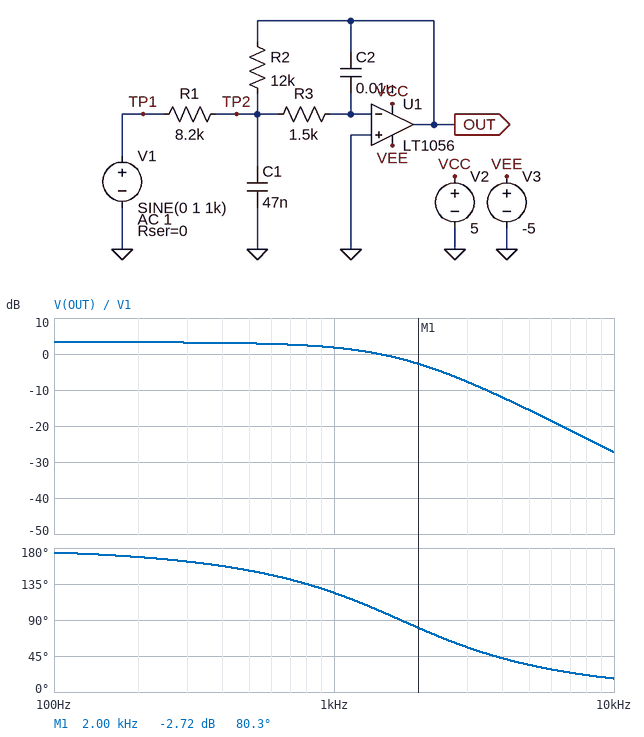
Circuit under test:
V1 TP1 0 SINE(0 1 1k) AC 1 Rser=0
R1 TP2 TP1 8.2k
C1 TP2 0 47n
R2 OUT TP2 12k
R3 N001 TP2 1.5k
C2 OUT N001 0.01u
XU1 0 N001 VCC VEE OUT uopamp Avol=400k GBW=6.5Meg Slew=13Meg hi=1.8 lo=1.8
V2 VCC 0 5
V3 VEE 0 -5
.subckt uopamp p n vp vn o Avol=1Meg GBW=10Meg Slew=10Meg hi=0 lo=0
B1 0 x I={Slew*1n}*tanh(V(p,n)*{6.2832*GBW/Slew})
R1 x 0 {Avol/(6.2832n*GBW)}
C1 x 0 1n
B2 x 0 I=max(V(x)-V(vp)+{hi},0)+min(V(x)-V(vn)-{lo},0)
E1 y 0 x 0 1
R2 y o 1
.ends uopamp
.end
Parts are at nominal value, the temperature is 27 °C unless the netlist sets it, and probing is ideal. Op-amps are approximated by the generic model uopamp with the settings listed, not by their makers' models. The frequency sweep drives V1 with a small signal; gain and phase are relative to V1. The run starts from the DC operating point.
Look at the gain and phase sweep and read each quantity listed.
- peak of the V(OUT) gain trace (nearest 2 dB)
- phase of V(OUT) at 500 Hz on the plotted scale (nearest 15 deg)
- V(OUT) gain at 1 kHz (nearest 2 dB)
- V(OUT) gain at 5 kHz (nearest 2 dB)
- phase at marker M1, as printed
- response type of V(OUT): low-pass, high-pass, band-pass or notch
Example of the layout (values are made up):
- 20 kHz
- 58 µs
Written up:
- 4 dB
- 150 deg
- 2 dB
- -16 dB
- 80.3 deg
- low-pass
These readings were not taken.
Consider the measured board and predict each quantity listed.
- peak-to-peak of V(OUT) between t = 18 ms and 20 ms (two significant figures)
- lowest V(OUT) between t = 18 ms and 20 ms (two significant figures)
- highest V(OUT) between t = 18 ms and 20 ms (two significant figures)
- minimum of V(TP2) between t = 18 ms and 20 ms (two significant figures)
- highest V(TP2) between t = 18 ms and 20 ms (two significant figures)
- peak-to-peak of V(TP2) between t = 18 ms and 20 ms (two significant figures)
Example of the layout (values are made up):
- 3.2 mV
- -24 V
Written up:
- 2.5 V
- -1.2 V
- 1.2 V
- -120 mV
- 120 mV
- 230 mV
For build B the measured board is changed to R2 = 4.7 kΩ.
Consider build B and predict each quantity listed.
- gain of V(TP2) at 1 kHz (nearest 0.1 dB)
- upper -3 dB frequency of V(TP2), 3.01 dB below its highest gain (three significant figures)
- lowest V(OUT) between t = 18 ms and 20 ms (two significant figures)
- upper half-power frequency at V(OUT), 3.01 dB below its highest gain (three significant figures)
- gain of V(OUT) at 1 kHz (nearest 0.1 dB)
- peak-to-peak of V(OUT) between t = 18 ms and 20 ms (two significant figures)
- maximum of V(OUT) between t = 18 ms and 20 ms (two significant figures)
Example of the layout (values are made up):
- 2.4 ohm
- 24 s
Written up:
- -25.1 dB
- 4.93 kHz
- -590 mV
- 3.05 kHz
- -4.6 dB
- 1.2 V
- 590 mV
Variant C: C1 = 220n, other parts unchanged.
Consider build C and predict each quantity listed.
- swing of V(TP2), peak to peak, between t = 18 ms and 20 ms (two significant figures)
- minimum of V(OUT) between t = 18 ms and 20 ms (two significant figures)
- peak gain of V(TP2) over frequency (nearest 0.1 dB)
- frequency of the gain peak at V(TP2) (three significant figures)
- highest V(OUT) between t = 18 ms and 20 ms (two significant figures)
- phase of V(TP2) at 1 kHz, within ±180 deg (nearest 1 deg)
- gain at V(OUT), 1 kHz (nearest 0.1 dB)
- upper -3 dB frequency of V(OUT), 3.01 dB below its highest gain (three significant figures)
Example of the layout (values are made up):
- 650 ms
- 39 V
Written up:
- 240 mV
- -1.3 V
- -17.1 dB
- 799 Hz
- 1.3 V
- -30 deg
- 2.2 dB
- 950 Hz
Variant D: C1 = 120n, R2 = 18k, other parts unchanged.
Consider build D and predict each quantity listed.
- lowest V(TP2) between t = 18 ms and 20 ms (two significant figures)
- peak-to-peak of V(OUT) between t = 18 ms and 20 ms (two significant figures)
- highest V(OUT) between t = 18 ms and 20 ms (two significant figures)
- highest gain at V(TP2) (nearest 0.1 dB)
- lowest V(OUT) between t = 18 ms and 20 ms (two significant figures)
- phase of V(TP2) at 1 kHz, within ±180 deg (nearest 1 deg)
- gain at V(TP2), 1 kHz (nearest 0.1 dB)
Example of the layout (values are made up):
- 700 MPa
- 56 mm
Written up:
- -140 mV
- 3.0 V
- 1.5 V
- -16.8 dB
- -1.5 V
- -11 deg
- -17.0 dB
